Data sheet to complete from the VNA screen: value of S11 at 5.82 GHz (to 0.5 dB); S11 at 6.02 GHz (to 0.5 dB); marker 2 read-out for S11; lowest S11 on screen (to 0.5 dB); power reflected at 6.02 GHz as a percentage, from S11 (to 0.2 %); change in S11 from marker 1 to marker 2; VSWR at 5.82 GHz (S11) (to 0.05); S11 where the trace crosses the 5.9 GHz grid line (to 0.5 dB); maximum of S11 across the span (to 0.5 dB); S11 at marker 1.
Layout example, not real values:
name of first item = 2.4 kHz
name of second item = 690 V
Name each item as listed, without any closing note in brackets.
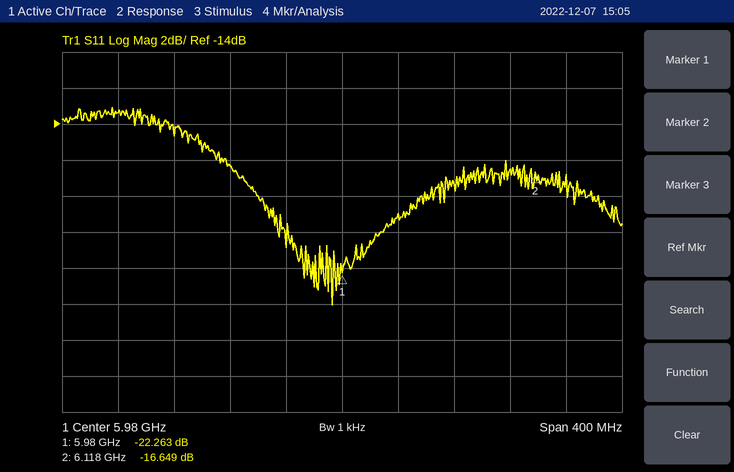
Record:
value of S11 at 5.82 GHz = -13.5 dB
S11 at 6.02 GHz = -19.0 dB
marker 2 read-out for S11 = -16.649 dB
lowest S11 on screen = -24.0 dB
power reflected at 6.02 GHz as a percentage, from S11 = 1.2 %
change in S11 from marker 1 to marker 2 = 5.614 dB
VSWR at 5.82 GHz (S11) = 1.55
S11 where the trace crosses the 5.9 GHz grid line = -16.5 dB
maximum of S11 across the span = -13.0 dB
S11 at marker 1 = -22.263 dB
